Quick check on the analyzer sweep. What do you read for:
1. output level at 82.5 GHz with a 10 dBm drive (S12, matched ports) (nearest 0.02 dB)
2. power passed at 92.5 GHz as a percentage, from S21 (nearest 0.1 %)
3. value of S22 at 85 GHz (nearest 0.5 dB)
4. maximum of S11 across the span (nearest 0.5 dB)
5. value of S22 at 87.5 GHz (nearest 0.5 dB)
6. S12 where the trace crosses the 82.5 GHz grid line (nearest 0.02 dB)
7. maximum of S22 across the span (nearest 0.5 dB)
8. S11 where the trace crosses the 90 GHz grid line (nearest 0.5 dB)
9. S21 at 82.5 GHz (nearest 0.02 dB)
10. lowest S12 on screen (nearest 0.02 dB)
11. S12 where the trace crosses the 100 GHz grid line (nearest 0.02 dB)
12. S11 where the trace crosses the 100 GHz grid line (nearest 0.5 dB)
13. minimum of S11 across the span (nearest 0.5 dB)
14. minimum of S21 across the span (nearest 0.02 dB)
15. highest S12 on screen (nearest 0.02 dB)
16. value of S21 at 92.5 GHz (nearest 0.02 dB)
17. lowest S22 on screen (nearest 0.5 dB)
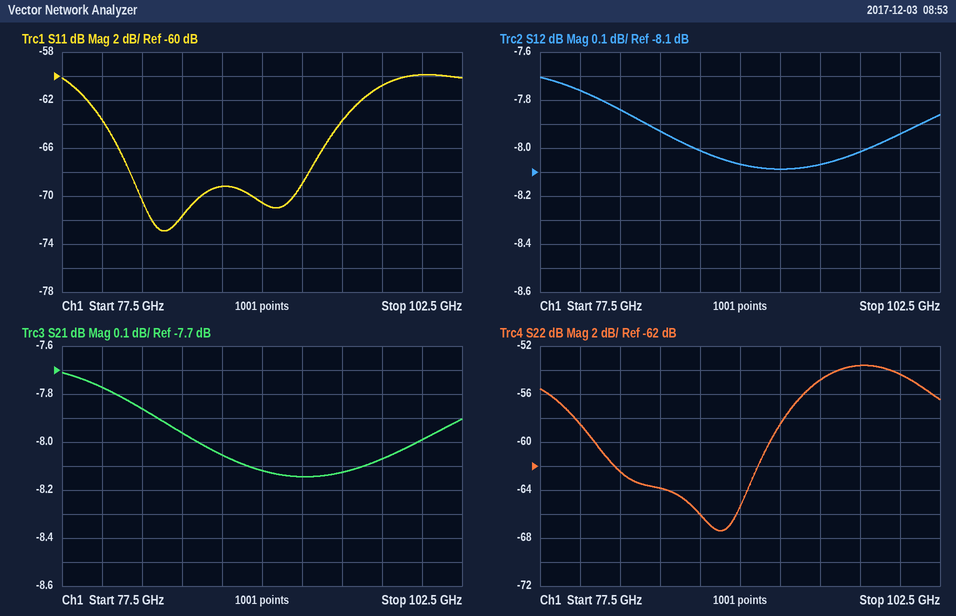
2.16 dBm
15.3 %
-64.0 dB
-60.0 dB
-66.0 dB
-7.84 dB
-53.5 dB
-70.5 dB
-7.86 dB
-8.08 dB
-7.94 dB
-60.0 dB
-73.0 dB
-8.14 dB
-7.70 dB
-8.14 dB
-67.5 dB
